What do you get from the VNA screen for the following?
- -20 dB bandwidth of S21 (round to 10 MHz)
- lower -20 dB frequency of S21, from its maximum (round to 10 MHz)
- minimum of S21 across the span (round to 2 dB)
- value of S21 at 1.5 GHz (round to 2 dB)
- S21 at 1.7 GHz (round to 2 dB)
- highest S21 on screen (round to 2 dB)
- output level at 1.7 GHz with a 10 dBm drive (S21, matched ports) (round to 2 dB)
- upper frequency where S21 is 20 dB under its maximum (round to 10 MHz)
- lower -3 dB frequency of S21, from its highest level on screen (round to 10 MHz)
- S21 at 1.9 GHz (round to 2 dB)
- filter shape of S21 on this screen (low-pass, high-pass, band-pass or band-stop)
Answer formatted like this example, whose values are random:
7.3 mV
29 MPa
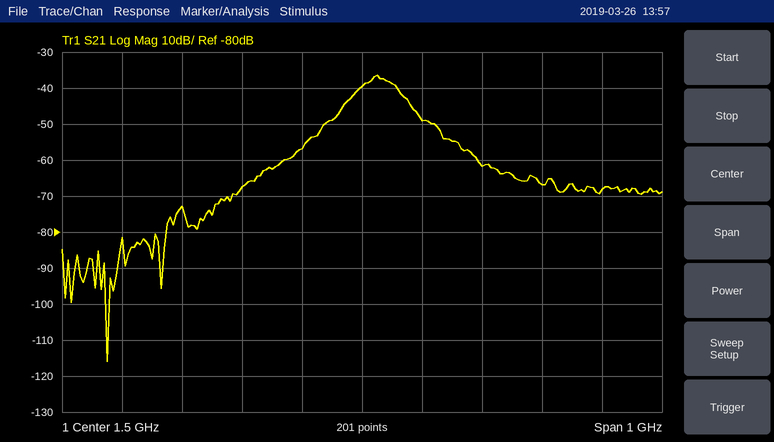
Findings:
260 MHz
1.40 GHz
-116 dB
-40 dB
-62 dB
-36 dB
-52 dBm
1.66 GHz
1.50 GHz
-68 dB
band-pass
